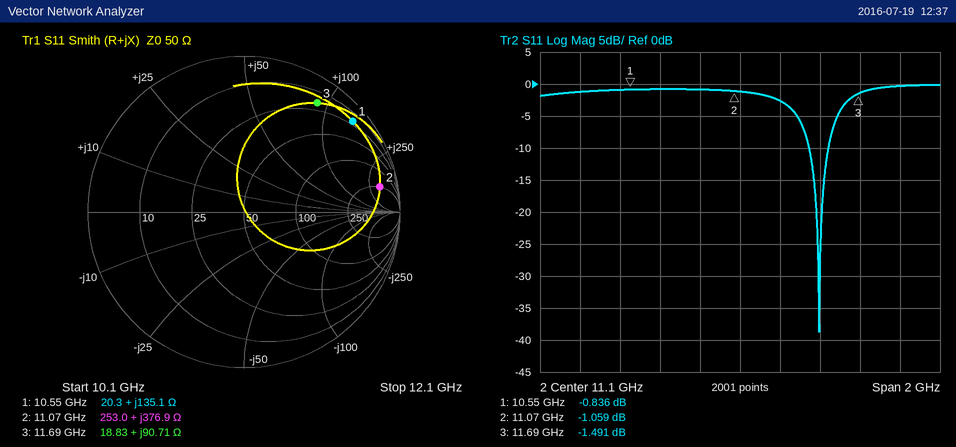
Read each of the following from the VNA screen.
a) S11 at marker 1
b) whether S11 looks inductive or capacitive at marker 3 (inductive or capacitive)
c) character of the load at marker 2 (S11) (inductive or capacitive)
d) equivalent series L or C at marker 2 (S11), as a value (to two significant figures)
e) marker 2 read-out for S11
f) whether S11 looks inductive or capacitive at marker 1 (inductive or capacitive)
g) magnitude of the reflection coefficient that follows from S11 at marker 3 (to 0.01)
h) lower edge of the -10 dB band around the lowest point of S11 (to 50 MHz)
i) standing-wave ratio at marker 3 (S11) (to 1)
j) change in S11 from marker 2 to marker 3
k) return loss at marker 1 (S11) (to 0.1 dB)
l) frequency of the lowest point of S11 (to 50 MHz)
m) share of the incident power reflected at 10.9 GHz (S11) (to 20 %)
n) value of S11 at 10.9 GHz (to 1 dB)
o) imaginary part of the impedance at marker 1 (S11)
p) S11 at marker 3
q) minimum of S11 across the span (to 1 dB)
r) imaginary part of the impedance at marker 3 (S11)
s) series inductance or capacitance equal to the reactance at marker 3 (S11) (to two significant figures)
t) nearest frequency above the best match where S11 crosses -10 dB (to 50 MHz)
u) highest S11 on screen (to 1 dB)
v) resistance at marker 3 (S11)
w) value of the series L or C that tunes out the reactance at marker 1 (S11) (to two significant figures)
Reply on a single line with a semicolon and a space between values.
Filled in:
-0.836 dB; inductive; inductive; 5.4 nH; -1.059 dB; inductive; 0.84; 11.45 GHz; 12; -0.432 dB; 0.8 dB; 11.50 GHz; 80 %; -1 dB; +135.1 Ω; -1.491 dB; -39 dB; +90.71 Ω; 1.2 nH; 11.55 GHz; 0 dB; 18.83 Ω; 110 fF
